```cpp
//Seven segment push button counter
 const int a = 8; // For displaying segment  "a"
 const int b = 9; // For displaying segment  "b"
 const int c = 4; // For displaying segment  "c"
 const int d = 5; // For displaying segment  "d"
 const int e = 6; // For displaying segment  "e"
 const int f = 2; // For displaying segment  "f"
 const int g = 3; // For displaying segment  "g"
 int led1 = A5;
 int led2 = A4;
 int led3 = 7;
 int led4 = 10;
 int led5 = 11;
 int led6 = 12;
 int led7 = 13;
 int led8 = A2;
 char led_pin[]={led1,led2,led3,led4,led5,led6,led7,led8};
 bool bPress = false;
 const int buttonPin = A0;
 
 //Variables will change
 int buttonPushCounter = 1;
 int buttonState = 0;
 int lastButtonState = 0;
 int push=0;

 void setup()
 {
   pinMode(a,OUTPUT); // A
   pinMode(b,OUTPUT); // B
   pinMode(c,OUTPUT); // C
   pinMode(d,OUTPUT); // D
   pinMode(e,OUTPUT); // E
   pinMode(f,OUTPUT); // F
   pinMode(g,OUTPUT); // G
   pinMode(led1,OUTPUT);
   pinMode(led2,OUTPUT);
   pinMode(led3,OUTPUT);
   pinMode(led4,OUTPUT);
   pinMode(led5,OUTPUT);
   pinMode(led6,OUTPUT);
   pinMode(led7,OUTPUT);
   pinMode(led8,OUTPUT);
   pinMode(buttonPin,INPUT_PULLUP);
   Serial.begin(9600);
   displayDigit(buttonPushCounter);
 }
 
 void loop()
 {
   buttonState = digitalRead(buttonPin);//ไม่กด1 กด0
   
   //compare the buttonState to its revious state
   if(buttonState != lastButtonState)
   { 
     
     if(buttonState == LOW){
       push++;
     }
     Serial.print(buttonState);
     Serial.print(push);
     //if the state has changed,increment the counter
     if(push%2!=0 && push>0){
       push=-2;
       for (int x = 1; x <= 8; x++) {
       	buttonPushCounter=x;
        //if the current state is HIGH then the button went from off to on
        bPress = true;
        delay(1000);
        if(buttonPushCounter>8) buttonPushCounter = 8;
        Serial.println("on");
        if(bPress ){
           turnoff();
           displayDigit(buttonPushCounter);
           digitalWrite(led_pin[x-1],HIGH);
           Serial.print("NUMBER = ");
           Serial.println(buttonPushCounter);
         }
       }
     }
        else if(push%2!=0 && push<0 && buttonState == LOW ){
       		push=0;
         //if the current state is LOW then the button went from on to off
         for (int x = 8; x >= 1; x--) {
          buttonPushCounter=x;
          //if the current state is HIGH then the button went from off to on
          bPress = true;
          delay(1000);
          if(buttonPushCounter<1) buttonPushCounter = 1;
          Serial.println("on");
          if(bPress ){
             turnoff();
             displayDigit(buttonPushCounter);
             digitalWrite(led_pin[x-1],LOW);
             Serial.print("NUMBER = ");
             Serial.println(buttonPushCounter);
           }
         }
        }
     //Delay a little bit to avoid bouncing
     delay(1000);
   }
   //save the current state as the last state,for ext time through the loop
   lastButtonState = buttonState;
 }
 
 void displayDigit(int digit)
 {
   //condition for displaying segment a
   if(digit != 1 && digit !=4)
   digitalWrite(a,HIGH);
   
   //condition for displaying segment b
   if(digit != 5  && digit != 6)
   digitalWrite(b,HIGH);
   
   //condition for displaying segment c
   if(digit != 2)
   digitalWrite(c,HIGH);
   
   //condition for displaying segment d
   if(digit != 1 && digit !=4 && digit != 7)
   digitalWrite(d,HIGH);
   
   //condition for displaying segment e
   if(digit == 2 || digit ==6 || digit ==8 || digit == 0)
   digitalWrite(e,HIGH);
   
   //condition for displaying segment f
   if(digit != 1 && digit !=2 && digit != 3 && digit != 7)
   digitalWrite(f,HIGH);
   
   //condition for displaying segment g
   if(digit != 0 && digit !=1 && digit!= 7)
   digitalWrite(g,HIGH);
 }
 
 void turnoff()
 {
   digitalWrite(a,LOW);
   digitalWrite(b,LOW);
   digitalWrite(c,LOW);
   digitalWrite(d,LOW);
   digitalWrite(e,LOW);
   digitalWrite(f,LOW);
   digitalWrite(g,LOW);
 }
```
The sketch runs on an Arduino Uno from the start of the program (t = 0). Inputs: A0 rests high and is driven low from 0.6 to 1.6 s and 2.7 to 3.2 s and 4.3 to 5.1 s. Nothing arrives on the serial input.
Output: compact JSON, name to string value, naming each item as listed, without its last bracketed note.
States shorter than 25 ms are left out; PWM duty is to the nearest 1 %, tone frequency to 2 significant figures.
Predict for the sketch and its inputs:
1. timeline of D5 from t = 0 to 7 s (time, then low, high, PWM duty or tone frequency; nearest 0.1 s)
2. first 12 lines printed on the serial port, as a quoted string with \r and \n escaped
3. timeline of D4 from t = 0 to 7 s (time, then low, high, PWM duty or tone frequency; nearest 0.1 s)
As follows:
{"timeline of D5 from t = 0 to 7 s": "0 s low; 3 s high; 5 s low; 6 s high", "first 12 lines printed on the serial port, as a quoted string with \\r and \\n escaped": "\"1001on\\r\\nNUMBER = 1\\r\\non\\r\\nNUMBER = 2\\r\\non\\r\\nNUMBER = 3\\r\\non\\r\\nNUMBER = 4\\r\\non\\r\\nNUMBER = 5\\r\\non\\r\\nNUMBER = 6\\r\\n\"", "timeline of D4 from t = 0 to 7 s": "0 s high; 3 s low; 4 s high"}
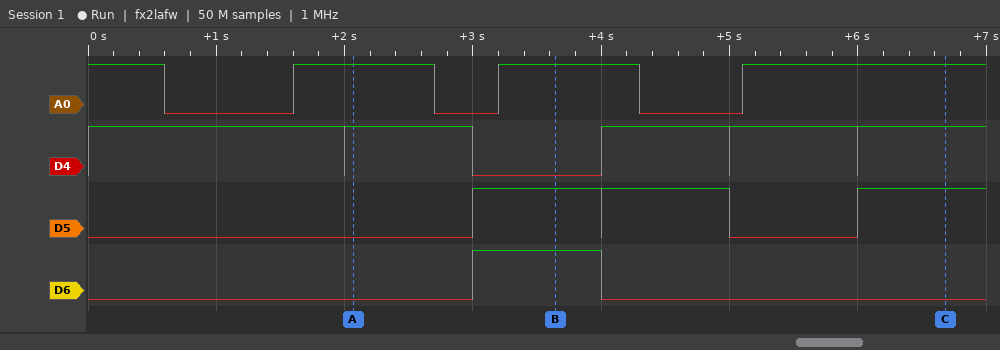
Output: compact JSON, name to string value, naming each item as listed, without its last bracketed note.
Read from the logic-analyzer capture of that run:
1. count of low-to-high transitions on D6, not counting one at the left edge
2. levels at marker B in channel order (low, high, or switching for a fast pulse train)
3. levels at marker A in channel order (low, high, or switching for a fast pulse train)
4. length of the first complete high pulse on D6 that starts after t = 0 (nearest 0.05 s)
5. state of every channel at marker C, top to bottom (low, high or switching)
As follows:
{"count of low-to-high transitions on D6, not counting one at the left edge": "1", "levels at marker B in channel order": "A0 high, D4 low, D5 high, D6 high", "levels at marker A in channel order": "A0 high, D4 high, D5 low, D6 low", "length of the first complete high pulse on D6 that starts after t = 0": "1.00 s", "state of every channel at marker C, top to bottom": "A0 high, D4 high, D5 high, D6 low"}
